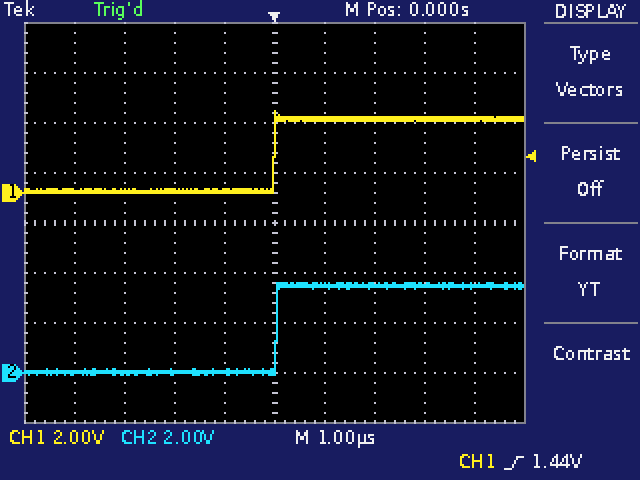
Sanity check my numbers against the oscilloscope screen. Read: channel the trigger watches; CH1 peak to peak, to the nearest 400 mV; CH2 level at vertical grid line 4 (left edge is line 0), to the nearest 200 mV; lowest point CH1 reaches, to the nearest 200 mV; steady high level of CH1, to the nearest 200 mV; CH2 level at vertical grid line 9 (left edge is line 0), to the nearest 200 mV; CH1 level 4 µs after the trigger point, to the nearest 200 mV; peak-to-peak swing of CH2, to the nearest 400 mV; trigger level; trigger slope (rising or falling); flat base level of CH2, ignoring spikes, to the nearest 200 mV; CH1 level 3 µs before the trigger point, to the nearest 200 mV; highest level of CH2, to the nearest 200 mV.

CH1
3.2 V
0.0 V
0.0 V
3.0 V
3.4 V
3.0 V
3.6 V
1.44 V
rising
0.0 V
0.0 V
3.6 V
